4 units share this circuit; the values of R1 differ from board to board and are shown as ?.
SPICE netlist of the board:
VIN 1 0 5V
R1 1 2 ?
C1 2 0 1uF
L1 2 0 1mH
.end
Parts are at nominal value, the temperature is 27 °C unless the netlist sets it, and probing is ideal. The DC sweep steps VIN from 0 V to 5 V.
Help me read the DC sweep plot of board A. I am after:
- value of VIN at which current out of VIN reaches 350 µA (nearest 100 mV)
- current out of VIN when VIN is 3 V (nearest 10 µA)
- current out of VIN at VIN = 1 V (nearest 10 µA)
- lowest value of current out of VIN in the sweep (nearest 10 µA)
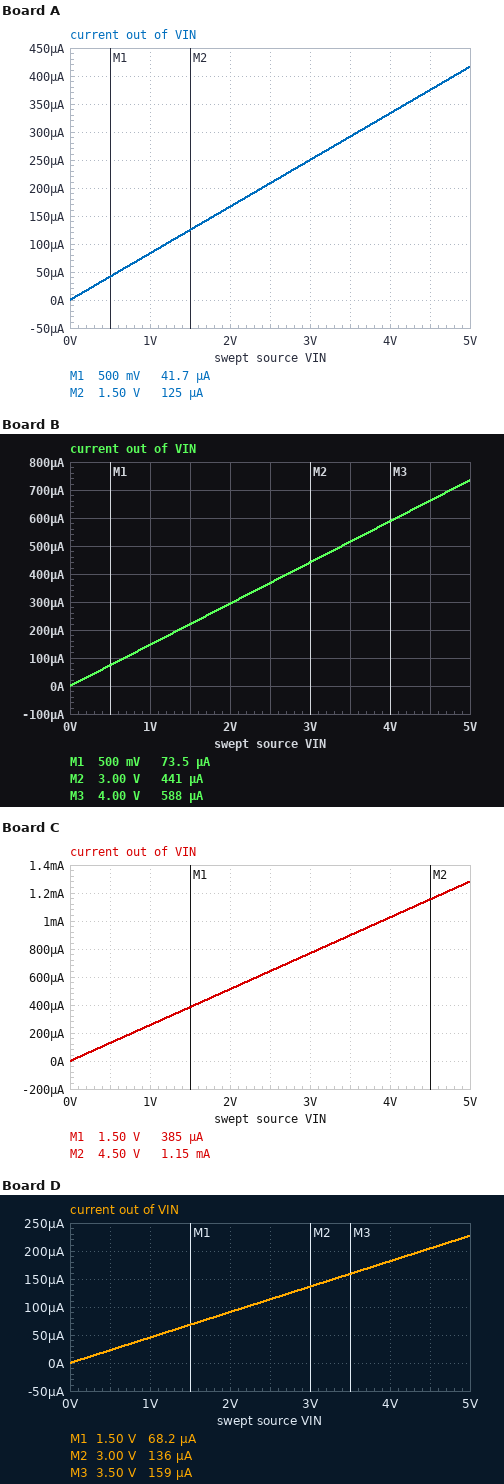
4.2 V
250 µA
80 µA
0 A
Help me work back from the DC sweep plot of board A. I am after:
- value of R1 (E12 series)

12 kΩ
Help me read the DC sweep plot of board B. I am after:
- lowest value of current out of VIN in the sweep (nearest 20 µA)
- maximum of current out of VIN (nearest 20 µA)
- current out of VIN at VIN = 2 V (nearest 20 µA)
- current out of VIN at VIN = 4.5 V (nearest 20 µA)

0 A
740 µA
300 µA
660 µA
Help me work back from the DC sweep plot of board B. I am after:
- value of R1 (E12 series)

6.8 kΩ
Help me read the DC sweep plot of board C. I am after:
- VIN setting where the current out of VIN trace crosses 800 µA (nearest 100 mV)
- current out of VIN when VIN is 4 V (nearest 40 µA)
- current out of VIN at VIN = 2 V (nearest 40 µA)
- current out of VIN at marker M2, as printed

3.1 V
1.04 mA
520 µA
1.15 mA
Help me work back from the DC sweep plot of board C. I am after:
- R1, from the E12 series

3.9 kΩ
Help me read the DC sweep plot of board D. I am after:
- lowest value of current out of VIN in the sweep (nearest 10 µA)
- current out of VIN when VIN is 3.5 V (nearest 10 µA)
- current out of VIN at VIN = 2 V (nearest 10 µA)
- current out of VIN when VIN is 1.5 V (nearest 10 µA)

0 A
160 µA
90 µA
70 µA
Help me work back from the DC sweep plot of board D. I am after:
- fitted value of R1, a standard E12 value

22 kΩ
